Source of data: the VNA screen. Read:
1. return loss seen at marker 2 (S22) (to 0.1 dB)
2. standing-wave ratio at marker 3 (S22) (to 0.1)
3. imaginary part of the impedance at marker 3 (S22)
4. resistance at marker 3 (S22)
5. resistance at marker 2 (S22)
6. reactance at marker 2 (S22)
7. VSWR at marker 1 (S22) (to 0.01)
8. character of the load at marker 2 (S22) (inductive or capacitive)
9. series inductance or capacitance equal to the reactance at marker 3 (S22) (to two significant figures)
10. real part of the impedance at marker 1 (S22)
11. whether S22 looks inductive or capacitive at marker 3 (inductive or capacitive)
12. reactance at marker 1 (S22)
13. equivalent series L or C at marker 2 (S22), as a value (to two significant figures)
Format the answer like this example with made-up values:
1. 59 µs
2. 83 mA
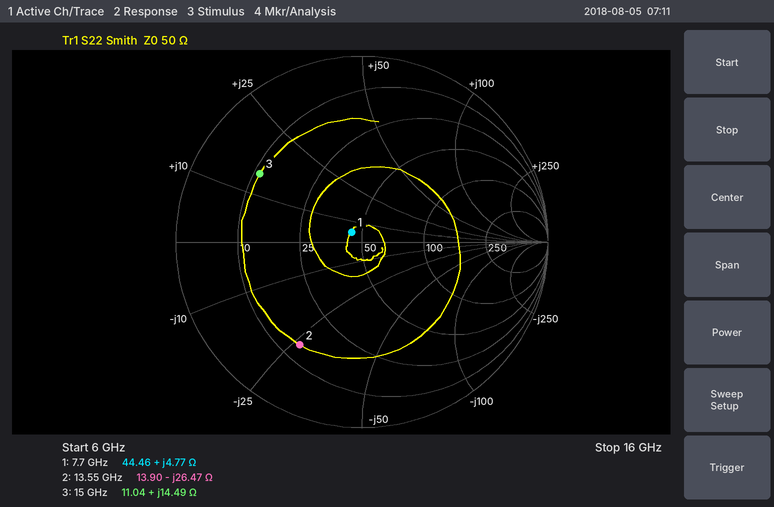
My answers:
1. 3.8 dB
2. 4.9
3. +14.49 Ω
4. 11.04 Ω
5. 13.90 Ω
6. -26.47 Ω
7. 1.17
8. capacitive
9. 150 pH
10. 44.46 Ω
11. inductive
12. +4.77 Ω
13. 440 fF
